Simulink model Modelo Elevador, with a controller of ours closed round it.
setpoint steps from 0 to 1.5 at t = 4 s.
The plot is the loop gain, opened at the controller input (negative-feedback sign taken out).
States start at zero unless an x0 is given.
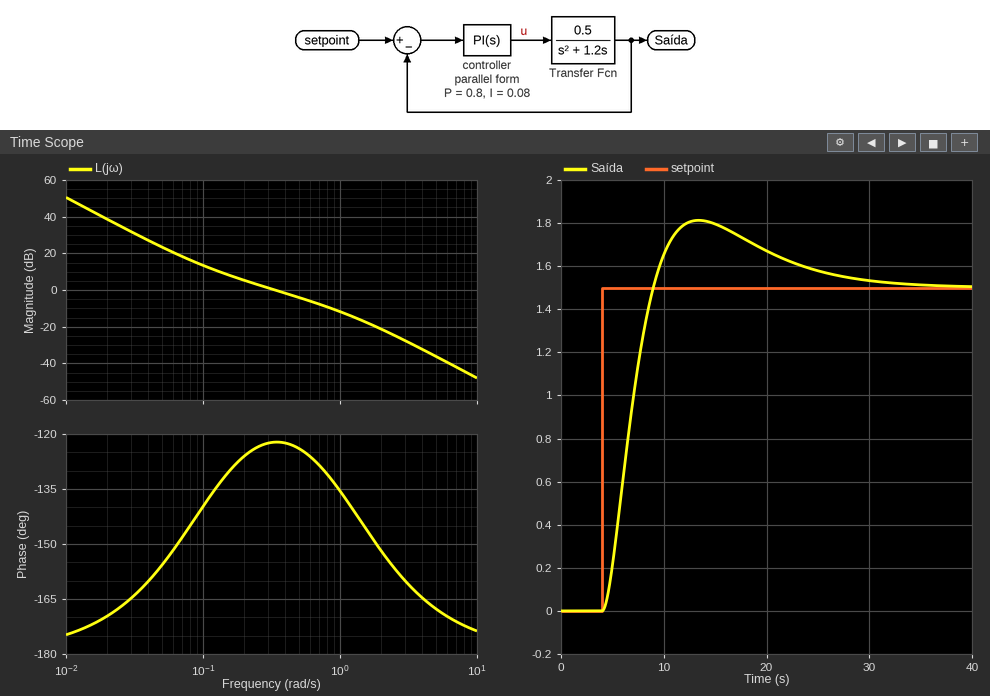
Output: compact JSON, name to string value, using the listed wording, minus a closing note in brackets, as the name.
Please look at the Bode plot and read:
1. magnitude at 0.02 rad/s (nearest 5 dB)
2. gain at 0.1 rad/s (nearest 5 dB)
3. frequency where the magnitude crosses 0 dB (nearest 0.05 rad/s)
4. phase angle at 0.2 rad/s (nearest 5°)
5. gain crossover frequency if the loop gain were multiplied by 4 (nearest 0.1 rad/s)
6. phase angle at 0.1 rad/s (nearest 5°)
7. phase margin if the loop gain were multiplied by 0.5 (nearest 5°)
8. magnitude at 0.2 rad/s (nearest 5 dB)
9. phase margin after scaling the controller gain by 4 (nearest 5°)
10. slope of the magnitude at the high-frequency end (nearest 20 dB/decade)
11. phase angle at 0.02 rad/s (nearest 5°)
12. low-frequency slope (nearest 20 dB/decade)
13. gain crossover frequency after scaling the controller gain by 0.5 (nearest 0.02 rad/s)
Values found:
{"magnitude at 0.02 rad/s": "40 dB", "gain at 0.1 rad/s": "15 dB", "frequency where the magnitude crosses 0 dB": "0.35 rad/s", "phase angle at 0.2 rad/s": "-125°", "gain crossover frequency if the loop gain were multiplied by 4": "1.0 rad/s", "phase angle at 0.1 rad/s": "-140°", "phase margin if the loop gain were multiplied by 0.5": "55°", "magnitude at 0.2 rad/s": "5 dB", "phase margin after scaling the controller gain by 4": "45°", "slope of the magnitude at the high-frequency end": "-40 dB/decade", "phase angle at 0.02 rad/s": "-170°", "low-frequency slope": "-40 dB/decade", "gain crossover frequency after scaling the controller gain by 0.5": "0.18 rad/s"}
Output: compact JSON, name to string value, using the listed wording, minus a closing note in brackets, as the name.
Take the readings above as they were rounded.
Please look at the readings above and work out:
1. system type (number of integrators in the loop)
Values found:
{"system type": "2"}
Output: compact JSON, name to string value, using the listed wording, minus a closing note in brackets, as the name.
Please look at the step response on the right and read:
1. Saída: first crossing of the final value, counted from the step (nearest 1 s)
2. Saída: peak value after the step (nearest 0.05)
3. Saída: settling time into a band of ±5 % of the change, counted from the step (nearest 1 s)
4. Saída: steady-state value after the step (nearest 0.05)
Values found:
{"Saída: first crossing of the final value, counted from the step": "5 s", "Saída: peak value after the step": "1.80", "Saída: settling time into a band of ±5 % of the change, counted from the step": "21 s", "Saída: steady-state value after the step": "1.50"}
